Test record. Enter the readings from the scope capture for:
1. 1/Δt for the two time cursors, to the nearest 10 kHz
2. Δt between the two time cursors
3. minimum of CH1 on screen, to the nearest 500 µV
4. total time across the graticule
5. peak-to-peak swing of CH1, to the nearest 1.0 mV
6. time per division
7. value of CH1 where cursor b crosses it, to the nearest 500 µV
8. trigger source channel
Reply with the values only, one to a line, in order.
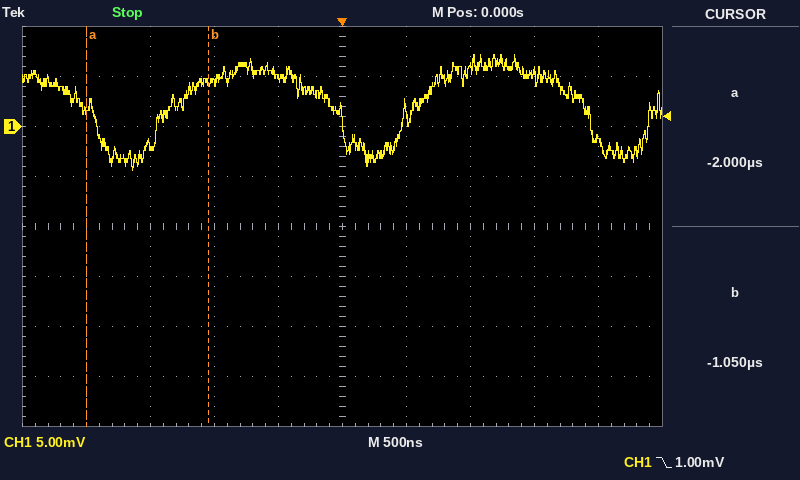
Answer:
1.05 MHz
950 ns
-4.5 mV
5 µs
12.0 mV
500 ns
4.5 mV
CH1
